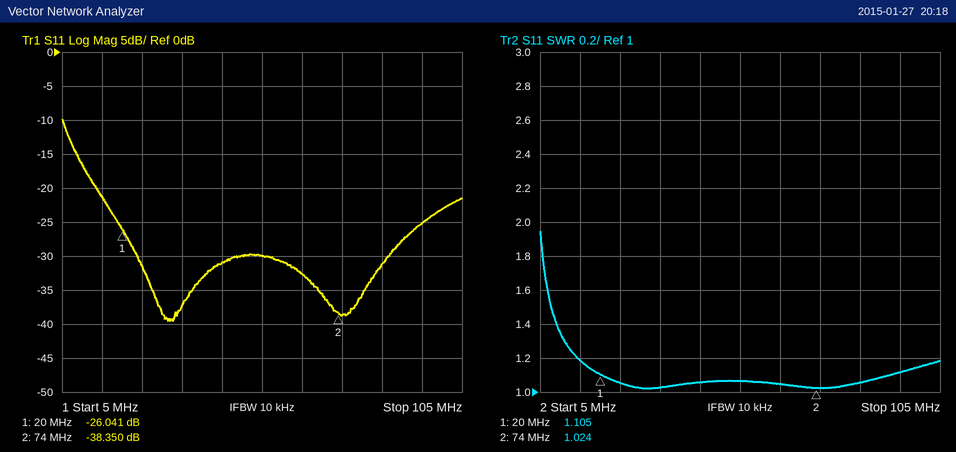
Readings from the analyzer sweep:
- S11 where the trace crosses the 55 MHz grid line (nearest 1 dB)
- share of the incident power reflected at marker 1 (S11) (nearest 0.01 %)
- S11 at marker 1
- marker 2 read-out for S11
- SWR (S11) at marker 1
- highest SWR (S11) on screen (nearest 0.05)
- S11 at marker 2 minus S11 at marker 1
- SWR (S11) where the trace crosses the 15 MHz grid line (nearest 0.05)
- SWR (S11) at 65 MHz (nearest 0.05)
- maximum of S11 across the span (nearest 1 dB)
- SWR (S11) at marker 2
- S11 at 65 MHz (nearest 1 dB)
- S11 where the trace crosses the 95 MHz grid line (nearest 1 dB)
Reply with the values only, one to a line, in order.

-30 dB
0.25 %
-26.041 dB
-38.350 dB
1.105
1.95
-12.309 dB
1.20
1.05
-10 dB
1.024
-33 dB
-25 dB
